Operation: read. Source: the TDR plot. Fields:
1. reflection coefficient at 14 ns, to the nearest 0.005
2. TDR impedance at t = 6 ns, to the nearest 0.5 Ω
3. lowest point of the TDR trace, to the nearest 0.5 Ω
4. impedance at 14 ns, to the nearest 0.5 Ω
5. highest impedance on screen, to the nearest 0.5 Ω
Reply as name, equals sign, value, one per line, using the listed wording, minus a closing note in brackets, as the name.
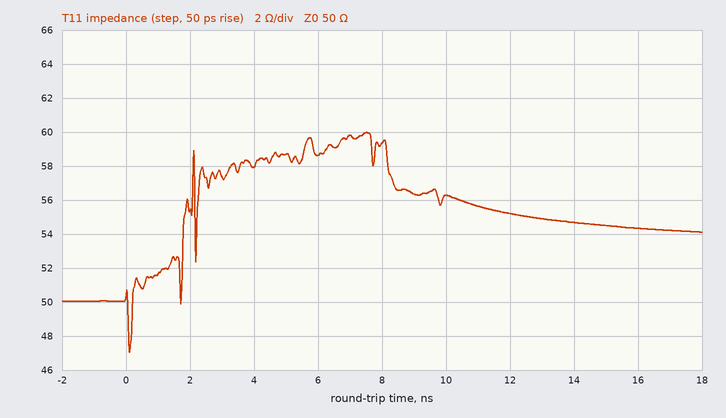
reflection coefficient at 14 ns, to the nearest 0.005 = +0.045
TDR impedance at t = 6 ns, to the nearest 0.5 Ω = 58.5 Ω
lowest point of the TDR trace, to the nearest 0.5 Ω = 47.0 Ω
impedance at 14 ns, to the nearest 0.5 Ω = 54.5 Ω
highest impedance on screen, to the nearest 0.5 Ω = 60.0 Ω
